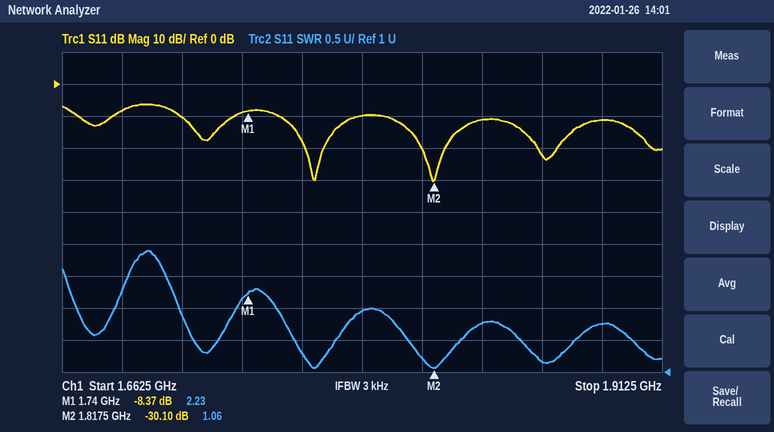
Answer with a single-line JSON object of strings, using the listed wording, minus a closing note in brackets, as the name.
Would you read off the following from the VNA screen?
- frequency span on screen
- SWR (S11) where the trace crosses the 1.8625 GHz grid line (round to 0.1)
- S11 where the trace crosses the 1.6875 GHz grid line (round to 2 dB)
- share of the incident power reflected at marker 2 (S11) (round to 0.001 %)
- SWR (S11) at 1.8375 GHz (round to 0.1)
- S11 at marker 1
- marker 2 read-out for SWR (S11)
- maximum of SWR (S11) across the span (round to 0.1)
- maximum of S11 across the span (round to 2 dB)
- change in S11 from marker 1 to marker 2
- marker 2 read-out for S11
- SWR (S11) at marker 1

{"frequency span on screen": "250 MHz", "SWR (S11) where the trace crosses the 1.8625 GHz grid line": "1.2", "S11 where the trace crosses the 1.6875 GHz grid line": "-8 dB", "share of the incident power reflected at marker 2 (S11)": "0.098 %", "SWR (S11) at 1.8375 GHz": "1.8", "S11 at marker 1": "-8.37 dB", "marker 2 read-out for SWR": "1.06", "maximum of SWR (S11) across the span": "2.9", "maximum of S11 across the span": "-6 dB", "change in S11 from marker 1 to marker 2": "-21.73 dB", "marker 2 read-out for S11": "-30.10 dB", "SWR (S11) at marker 1": "2.23"}
